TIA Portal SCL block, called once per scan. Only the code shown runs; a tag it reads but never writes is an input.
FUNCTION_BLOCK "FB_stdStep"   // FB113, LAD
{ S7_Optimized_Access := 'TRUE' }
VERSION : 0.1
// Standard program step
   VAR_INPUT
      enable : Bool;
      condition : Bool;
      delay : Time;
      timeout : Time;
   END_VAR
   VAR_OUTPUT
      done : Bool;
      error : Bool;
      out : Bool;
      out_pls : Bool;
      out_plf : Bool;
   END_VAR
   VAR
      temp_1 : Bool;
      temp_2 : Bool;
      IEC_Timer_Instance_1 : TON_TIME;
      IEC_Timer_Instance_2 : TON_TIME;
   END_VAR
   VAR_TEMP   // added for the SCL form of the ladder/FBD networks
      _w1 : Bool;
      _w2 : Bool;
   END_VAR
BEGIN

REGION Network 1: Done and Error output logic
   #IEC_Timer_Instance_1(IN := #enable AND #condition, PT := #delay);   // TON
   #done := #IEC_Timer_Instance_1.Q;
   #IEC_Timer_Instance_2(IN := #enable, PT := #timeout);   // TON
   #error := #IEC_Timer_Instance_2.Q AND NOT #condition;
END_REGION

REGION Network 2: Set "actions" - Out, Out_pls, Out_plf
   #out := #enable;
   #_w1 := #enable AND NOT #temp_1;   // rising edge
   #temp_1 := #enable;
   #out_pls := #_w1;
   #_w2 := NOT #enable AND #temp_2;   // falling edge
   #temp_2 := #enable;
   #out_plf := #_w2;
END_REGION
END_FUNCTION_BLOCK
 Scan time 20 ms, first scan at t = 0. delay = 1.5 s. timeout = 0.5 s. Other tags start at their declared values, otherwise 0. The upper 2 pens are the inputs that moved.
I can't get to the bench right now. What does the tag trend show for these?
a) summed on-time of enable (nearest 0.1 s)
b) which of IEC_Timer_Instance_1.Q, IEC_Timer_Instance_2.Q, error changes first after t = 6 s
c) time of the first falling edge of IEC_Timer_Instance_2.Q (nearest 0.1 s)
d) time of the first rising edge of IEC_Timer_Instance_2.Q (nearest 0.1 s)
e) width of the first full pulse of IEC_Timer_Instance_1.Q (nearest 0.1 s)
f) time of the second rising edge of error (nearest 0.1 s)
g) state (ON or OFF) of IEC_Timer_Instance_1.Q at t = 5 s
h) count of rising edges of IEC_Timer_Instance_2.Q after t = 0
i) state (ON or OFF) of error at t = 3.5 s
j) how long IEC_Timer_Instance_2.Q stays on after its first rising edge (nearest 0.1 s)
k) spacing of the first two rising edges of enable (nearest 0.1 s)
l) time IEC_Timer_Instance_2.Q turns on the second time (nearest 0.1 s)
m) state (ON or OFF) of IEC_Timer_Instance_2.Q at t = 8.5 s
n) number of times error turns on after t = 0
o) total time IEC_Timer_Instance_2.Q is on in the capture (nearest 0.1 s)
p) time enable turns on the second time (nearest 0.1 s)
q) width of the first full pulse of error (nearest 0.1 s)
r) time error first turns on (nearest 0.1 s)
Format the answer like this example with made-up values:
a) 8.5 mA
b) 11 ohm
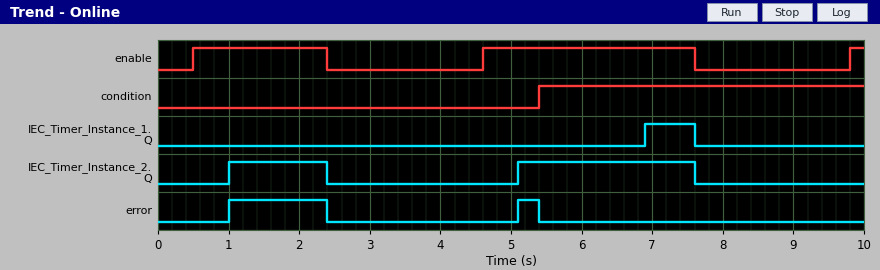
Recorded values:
a) 5.1 s
b) IEC_Timer_Instance_1.Q
c) 2.4 s
d) 1.0 s
e) 0.7 s
f) 5.1 s
g) OFF
h) 2
i) OFF
j) 1.4 s
k) 4.1 s
l) 5.1 s
m) OFF
n) 2
o) 3.9 s
p) 4.6 s
q) 1.4 s
r) 1.0 s
